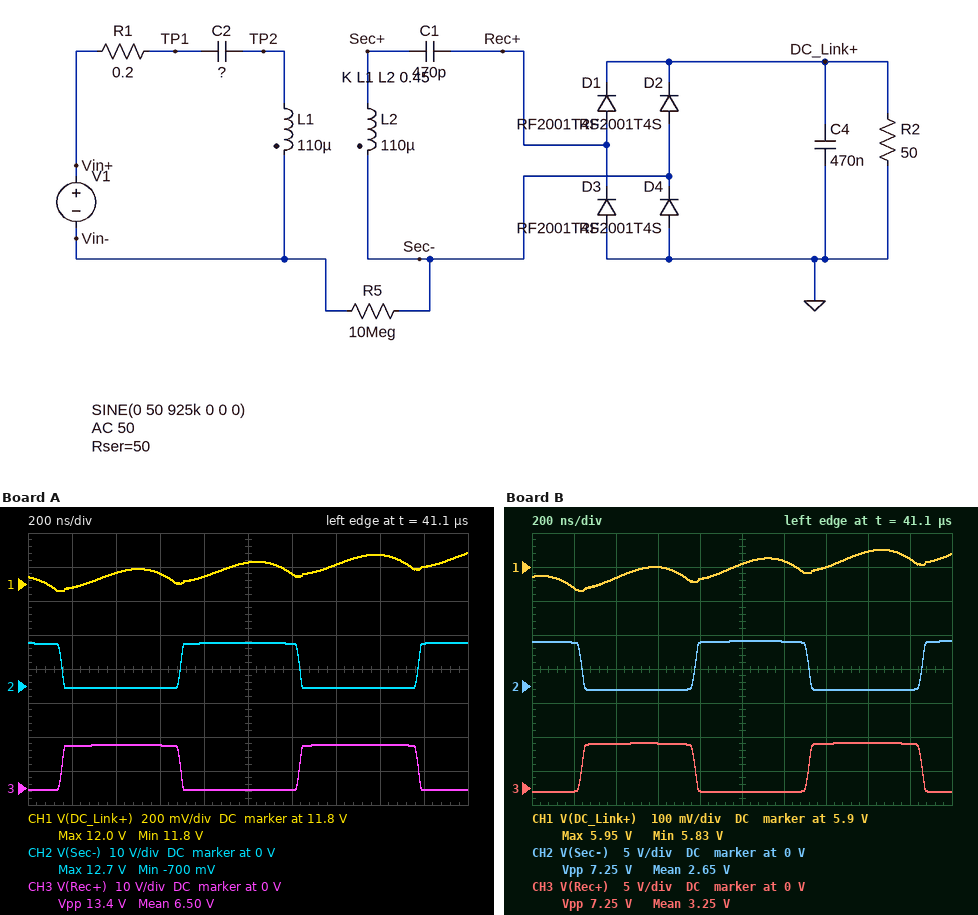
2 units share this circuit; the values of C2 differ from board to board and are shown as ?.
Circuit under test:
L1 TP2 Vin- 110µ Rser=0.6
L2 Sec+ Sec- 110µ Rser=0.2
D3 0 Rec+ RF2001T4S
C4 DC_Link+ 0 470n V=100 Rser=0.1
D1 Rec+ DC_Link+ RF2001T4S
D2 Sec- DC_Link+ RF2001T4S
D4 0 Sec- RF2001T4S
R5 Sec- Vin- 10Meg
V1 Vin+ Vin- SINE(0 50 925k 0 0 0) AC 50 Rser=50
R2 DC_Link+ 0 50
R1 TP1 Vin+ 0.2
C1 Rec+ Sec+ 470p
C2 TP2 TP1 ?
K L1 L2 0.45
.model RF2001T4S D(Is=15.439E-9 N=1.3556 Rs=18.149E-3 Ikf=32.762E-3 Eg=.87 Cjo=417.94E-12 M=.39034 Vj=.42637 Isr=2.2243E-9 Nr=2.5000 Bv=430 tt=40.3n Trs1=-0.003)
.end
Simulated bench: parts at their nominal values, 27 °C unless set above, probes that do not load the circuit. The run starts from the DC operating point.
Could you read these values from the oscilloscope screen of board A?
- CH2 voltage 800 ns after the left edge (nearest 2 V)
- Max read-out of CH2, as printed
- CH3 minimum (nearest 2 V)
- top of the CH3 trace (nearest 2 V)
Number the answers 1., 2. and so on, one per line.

1. 12 V
2. 12.7 V
3. 0 V
4. 12 V
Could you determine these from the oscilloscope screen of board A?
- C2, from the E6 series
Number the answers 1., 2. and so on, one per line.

1. 680 pF
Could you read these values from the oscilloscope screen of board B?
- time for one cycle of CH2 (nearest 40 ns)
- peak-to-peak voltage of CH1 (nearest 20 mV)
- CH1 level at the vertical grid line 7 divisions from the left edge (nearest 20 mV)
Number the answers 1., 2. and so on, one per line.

1. 1.08 µs
2. 120 mV
3. 5.90 V
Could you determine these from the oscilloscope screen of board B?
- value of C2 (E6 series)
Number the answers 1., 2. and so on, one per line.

1. 1.5 nF
